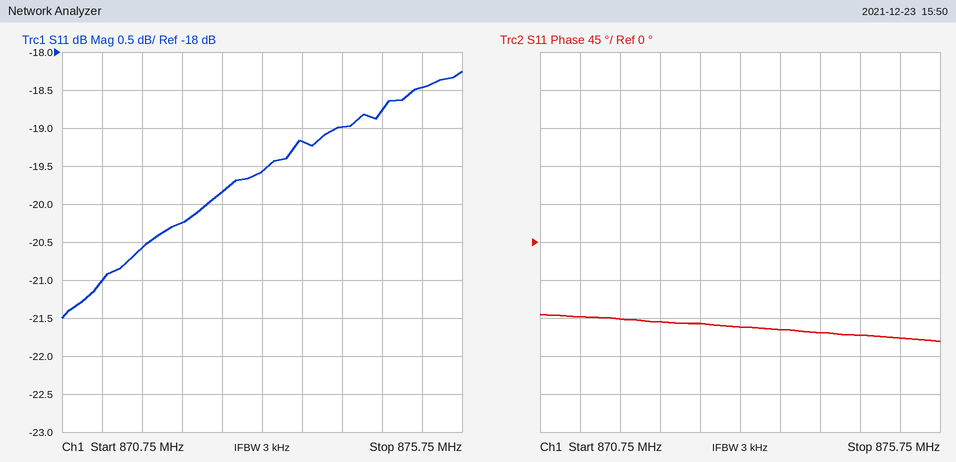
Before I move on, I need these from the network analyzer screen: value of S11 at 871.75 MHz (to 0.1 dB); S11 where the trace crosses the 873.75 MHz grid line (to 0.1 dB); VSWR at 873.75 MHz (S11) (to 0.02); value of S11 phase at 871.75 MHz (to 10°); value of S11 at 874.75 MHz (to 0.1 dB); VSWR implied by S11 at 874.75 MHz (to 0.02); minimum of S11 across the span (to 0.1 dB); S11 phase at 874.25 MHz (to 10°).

-20.6 dB
-19.2 dB
1.24
-90°
-18.8 dB
1.26
-21.5 dB
-110°
